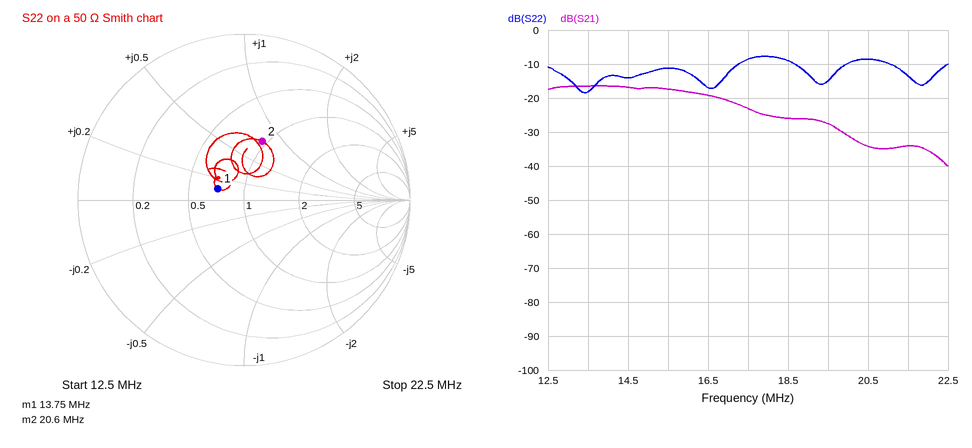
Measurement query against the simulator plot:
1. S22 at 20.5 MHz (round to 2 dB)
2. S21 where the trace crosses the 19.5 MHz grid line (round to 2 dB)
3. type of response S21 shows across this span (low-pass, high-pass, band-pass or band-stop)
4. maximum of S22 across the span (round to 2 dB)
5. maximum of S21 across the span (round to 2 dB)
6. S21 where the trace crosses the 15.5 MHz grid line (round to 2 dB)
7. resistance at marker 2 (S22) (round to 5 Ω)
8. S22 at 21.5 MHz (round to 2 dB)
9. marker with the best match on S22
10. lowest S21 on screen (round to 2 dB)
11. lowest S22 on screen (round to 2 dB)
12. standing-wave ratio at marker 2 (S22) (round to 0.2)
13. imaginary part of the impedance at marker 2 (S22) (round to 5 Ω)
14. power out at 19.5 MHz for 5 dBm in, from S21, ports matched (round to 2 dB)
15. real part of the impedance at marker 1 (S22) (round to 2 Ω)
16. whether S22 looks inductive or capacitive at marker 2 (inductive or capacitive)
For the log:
-8 dB
-28 dB
low-pass
-8 dB
-16 dB
-18 dB
45 Ω
-14 dB
marker 1
-40 dB
-18 dB
2.2
+40 Ω
-22 dBm
36 Ω
inductive
